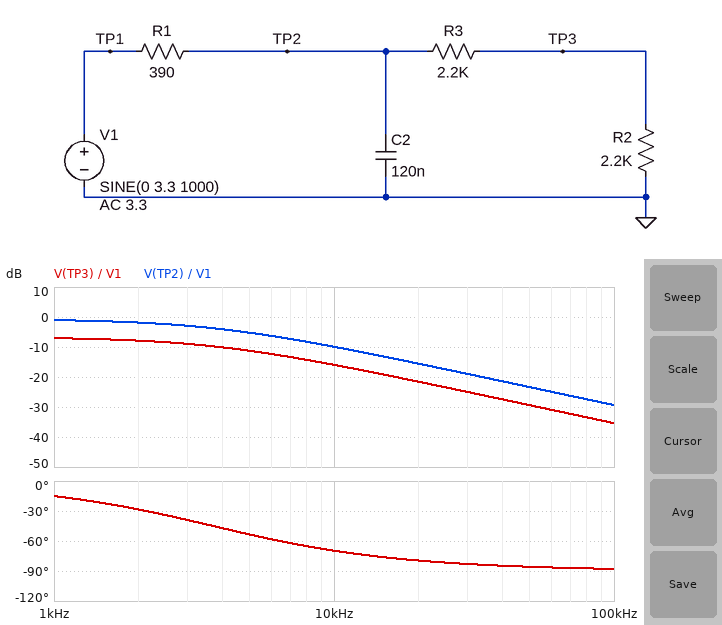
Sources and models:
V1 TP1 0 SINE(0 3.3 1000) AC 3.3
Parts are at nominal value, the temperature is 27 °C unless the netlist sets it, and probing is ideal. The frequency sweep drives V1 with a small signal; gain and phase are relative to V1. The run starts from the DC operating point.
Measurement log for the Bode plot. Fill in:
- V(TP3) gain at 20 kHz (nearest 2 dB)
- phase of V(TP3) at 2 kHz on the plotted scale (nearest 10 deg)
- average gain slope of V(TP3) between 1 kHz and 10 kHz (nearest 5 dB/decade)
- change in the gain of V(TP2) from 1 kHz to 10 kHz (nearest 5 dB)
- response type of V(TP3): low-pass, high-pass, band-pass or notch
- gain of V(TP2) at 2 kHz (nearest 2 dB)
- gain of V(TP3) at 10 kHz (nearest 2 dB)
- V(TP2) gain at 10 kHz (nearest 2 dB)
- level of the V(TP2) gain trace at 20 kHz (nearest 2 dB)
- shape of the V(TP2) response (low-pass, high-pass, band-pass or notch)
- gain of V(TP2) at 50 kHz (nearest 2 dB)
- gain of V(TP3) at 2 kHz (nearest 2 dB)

-22 dB
-30 deg
-10 dB/decade
-10 dB
low-pass
-2 dB
-16 dB
-10 dB
-16 dB
low-pass
-24 dB
-8 dB
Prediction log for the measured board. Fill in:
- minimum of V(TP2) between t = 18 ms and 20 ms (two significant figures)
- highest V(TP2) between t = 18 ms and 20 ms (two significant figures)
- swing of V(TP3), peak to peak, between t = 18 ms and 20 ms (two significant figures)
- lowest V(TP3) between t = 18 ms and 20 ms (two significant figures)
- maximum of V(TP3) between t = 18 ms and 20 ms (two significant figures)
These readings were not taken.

-2.9 V
2.9 V
2.9 V
-1.5 V
1.5 V
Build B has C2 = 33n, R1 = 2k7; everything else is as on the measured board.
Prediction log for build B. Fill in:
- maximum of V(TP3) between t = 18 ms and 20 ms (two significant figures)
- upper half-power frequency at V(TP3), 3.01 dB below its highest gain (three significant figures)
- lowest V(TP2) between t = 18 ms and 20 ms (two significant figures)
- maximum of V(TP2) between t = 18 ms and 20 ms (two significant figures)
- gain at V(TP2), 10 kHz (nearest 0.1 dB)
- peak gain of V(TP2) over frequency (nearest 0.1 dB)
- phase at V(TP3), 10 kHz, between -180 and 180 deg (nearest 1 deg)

970 mV
2.88 kHz
-1.9 V
1.9 V
-15.3 dB
-4.2 dB
-74 deg
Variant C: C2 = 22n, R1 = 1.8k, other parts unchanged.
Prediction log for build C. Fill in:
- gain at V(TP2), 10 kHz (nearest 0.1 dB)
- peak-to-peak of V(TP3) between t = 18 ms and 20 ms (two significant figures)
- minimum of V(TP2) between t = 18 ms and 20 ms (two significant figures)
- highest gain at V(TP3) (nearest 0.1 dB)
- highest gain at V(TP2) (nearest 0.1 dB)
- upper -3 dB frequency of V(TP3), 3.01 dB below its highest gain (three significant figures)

-9.1 dB
2.3 V
-2.3 V
-9.0 dB
-3.0 dB
5.66 kHz
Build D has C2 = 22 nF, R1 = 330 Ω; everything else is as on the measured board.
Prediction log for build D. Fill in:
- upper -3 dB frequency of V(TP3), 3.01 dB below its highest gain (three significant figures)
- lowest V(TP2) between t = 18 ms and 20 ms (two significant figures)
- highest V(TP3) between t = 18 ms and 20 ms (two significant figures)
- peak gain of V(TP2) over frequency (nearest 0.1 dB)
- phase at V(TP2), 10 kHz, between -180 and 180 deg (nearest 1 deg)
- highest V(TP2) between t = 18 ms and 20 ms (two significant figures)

23.6 kHz
-3.1 V
1.5 V
-0.6 dB
-23 deg
3.1 V
